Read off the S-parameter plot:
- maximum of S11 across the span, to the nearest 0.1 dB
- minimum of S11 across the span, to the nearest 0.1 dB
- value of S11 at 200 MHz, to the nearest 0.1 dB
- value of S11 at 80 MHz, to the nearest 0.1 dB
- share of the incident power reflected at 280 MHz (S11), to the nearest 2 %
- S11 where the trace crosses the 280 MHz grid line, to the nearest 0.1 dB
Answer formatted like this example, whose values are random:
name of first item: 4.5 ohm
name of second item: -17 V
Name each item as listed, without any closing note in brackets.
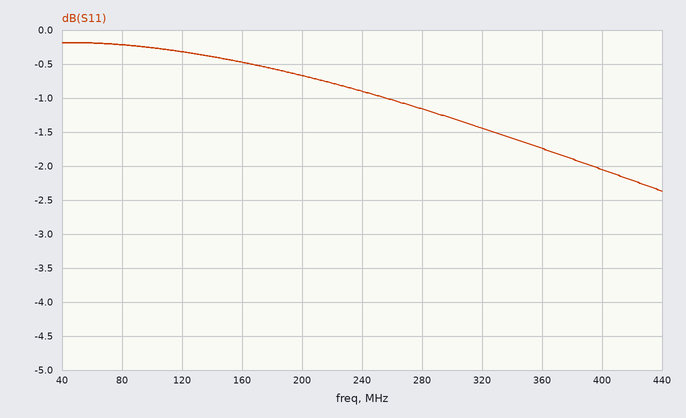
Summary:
maximum of S11 across the span, to the nearest 0.1 dB: -0.2 dB
minimum of S11 across the span, to the nearest 0.1 dB: -2.4 dB
value of S11 at 200 MHz, to the nearest 0.1 dB: -0.7 dB
value of S11 at 80 MHz, to the nearest 0.1 dB: -0.2 dB
share of the incident power reflected at 280 MHz (S11), to the nearest 2 %: 76 %
S11 where the trace crosses the 280 MHz grid line, to the nearest 0.1 dB: -1.2 dB
